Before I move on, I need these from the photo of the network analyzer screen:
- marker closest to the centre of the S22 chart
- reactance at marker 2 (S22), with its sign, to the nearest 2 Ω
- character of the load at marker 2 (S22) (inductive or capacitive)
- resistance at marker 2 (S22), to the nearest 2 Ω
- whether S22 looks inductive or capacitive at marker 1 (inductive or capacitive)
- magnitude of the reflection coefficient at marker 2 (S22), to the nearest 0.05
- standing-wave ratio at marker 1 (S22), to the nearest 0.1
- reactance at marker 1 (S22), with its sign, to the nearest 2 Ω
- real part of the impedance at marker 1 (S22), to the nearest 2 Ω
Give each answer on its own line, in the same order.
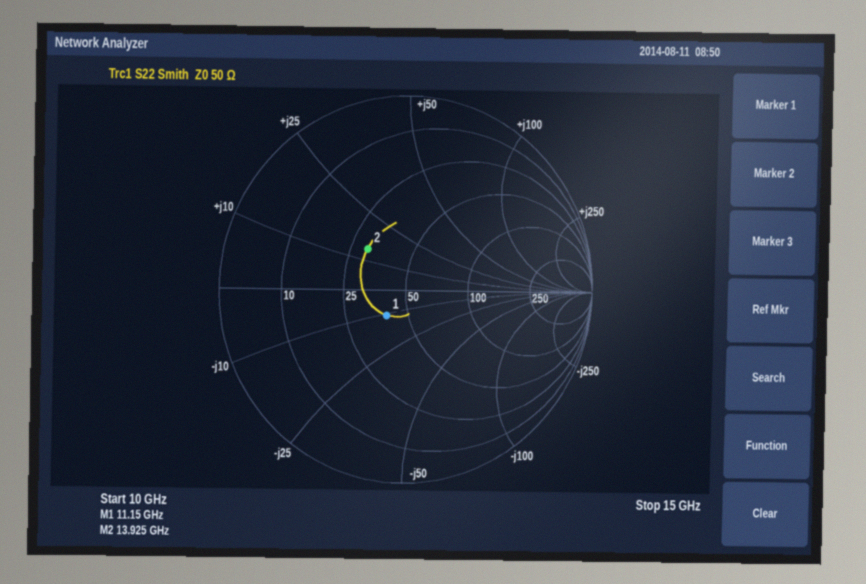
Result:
marker 1
+14 Ω
inductive
30 Ω
capacitive
0.30
1.4
-10 Ω
40 Ω
